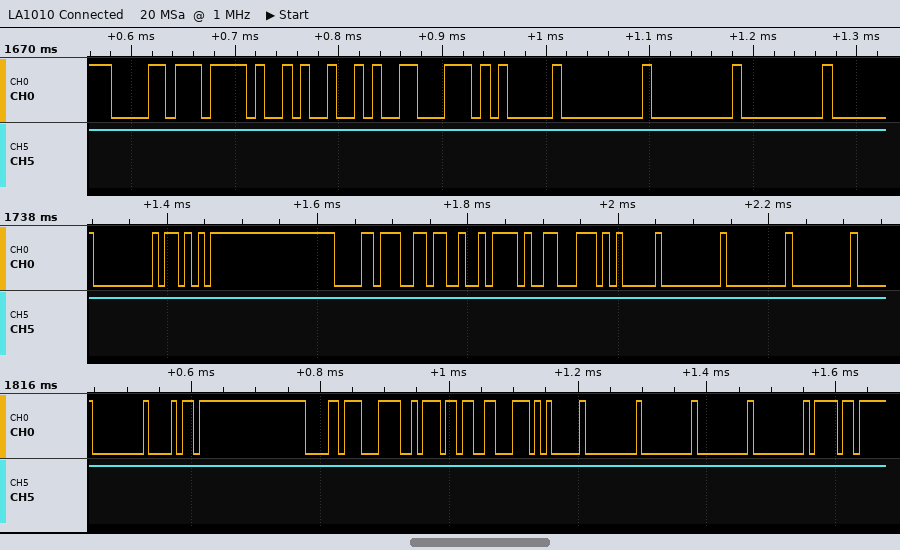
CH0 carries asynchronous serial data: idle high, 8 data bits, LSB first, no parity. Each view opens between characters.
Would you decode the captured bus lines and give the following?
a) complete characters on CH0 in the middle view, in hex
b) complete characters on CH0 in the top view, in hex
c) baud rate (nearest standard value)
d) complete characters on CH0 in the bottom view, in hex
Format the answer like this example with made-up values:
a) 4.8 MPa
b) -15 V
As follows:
a) 00, AB, D8, 36, 7A, C6, 05, 00, 00, 00
b) D8, 2F, 49, C6, 05, 00, 00, 00
c) 115200 baud
d) 00, 68, D8, 3C, B7, C6, 05, 00, 00, 00, 00, 6F
